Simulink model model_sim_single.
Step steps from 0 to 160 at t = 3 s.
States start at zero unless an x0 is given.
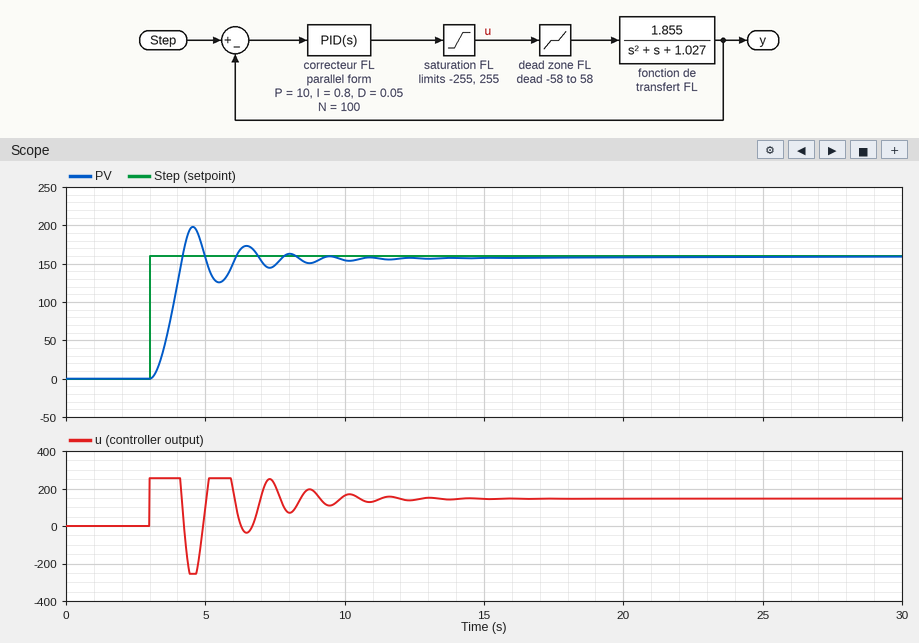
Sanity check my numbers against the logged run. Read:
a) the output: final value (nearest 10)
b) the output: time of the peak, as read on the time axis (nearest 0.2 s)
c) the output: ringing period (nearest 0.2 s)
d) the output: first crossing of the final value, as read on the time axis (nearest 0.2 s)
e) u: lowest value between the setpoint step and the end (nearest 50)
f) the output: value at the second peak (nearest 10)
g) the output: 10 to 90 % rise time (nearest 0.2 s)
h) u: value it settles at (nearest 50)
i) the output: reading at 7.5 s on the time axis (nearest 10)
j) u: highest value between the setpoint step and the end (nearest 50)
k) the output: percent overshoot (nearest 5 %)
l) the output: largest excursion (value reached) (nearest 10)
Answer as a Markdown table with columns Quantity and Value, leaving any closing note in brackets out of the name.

| Quantity | Value |
|---|---|
| the output: final value | 160 |
| the output: time of the peak, as read on the time axis | 4.6 s |
| the output: ringing period | 2.0 s |
| the output: first crossing of the final value, as read on the time axis | 4.2 s |
| u: lowest value between the setpoint step and the end | -250 |
| the output: value at the second peak | 170 |
| the output: 10 to 90 % rise time | 0.8 s |
| u: value it settles at | 150 |
| the output: reading at 7.5 s on the time axis | 150 |
| u: highest value between the setpoint step and the end | 250 |
| the output: percent overshoot | 25 % |
| the output: largest excursion (value reached) | 200 |
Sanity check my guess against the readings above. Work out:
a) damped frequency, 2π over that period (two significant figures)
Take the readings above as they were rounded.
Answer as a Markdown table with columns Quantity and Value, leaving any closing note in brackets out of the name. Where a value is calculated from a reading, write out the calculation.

| Quantity | Value |
|---|---|
| damped frequency, 2π over that period | 2π / 2 = 3.1 rad/s |
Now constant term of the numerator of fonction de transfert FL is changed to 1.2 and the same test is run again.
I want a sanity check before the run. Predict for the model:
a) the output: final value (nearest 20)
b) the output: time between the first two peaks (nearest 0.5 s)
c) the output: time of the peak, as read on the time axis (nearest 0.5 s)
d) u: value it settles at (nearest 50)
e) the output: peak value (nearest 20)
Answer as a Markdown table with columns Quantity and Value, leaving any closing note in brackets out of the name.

| Quantity | Value |
|---|---|
| the output: final value | 160 |
| the output: time between the first two peaks | 2.5 s |
| the output: time of the peak, as read on the time axis | 5.0 s |
| u: value it settles at | 200 |
| the output: peak value | 180 |
